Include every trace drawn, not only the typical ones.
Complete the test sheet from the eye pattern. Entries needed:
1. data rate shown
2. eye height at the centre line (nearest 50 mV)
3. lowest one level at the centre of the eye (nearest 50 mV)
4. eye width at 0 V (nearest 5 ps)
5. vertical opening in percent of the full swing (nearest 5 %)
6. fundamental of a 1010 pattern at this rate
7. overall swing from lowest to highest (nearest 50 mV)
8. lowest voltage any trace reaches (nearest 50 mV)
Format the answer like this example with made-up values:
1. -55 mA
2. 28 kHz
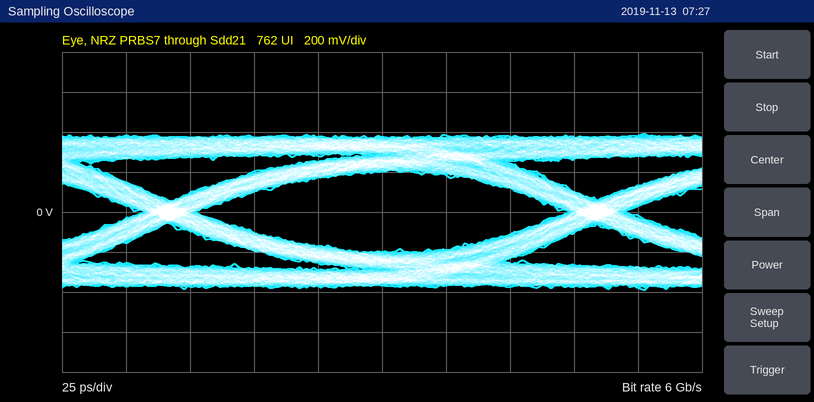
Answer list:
1. 6 Gb/s
2. 400 mV
3. 200 mV
4. 145 ps
5. 50 %
6. 3 GHz
7. 800 mV
8. -400 mV
